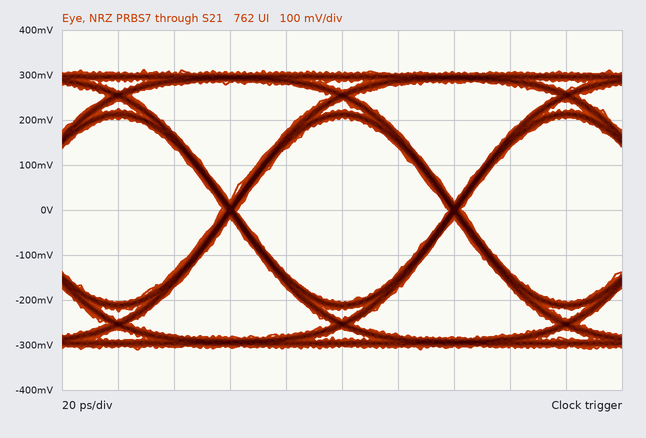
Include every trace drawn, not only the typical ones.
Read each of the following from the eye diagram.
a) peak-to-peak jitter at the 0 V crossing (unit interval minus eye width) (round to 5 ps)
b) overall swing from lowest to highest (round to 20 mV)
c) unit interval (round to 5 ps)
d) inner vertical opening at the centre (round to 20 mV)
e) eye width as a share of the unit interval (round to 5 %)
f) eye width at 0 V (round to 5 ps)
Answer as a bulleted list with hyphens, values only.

- 5 ps
- 620 mV
- 80 ps
- 420 mV
- 95 %
- 75 ps
